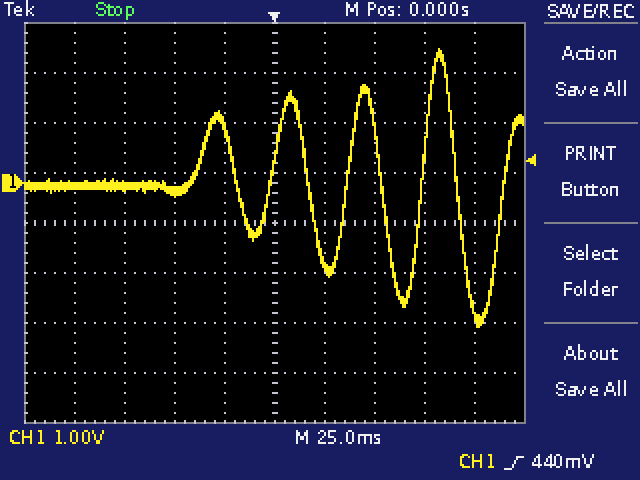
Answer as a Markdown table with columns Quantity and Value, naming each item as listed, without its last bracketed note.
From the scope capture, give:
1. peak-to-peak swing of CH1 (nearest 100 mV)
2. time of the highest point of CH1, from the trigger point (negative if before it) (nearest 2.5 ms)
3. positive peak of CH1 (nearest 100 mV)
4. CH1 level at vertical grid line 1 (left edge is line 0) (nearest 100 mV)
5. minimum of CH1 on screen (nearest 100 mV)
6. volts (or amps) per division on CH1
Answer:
| Quantity | Value |
|---|---|
| peak-to-peak swing of CH1 | 5.6 V |
| time of the highest point of CH1, from the trigger point (negative if before it) | +82.5 ms |
| positive peak of CH1 | 2.7 V |
| CH1 level at vertical grid line 1 (left edge is line 0) | -100 mV |
| minimum of CH1 on screen | -2.9 V |
| volts (or amps) per division on CH1 | 1 V |
